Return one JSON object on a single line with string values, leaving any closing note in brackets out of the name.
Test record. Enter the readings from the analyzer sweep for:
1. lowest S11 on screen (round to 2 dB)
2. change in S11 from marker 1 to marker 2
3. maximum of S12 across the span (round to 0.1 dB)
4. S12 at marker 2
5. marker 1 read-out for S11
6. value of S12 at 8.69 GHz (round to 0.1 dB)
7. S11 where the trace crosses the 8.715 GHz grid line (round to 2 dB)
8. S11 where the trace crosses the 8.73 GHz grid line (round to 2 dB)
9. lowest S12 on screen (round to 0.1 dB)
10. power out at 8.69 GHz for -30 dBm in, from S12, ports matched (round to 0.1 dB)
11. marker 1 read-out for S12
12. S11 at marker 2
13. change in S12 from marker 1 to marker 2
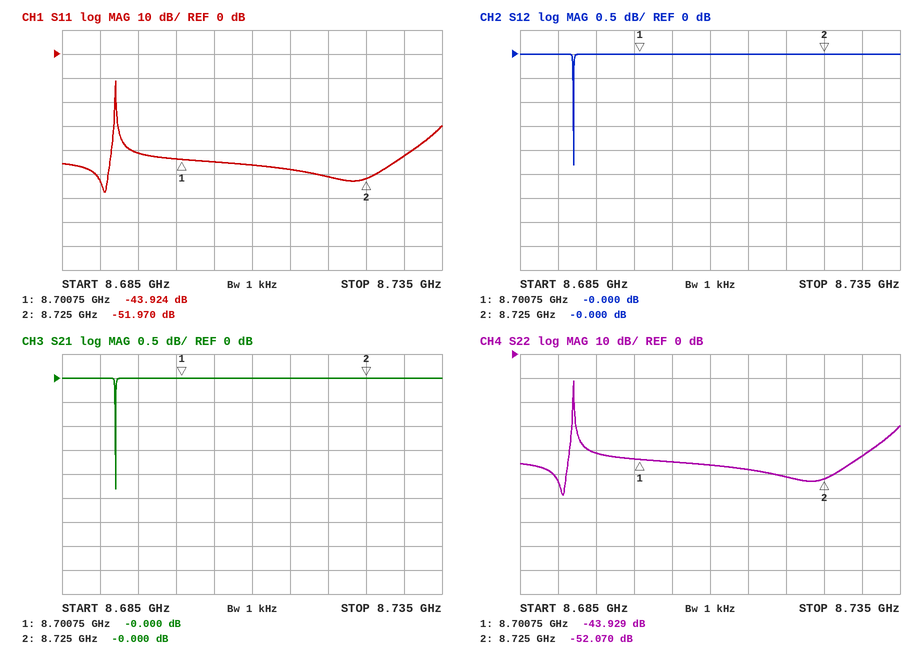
{"lowest S11 on screen": "-58 dB", "change in S11 from marker 1 to marker 2": "-8.046 dB", "maximum of S12 across the span": "0.0 dB", "S12 at marker 2": "-0.000 dB", "marker 1 read-out for S11": "-43.924 dB", "value of S12 at 8.69 GHz": "0.0 dB", "S11 where the trace crosses the 8.715 GHz grid line": "-48 dB", "S11 where the trace crosses the 8.73 GHz grid line": "-42 dB", "lowest S12 on screen": "-2.3 dB", "power out at 8.69 GHz for -30 dBm in, from S12, ports matched": "-30.0 dBm", "marker 1 read-out for S12": "-0.000 dB", "S11 at marker 2": "-51.970 dB", "change in S12 from marker 1 to marker 2": "0.000 dB"}
